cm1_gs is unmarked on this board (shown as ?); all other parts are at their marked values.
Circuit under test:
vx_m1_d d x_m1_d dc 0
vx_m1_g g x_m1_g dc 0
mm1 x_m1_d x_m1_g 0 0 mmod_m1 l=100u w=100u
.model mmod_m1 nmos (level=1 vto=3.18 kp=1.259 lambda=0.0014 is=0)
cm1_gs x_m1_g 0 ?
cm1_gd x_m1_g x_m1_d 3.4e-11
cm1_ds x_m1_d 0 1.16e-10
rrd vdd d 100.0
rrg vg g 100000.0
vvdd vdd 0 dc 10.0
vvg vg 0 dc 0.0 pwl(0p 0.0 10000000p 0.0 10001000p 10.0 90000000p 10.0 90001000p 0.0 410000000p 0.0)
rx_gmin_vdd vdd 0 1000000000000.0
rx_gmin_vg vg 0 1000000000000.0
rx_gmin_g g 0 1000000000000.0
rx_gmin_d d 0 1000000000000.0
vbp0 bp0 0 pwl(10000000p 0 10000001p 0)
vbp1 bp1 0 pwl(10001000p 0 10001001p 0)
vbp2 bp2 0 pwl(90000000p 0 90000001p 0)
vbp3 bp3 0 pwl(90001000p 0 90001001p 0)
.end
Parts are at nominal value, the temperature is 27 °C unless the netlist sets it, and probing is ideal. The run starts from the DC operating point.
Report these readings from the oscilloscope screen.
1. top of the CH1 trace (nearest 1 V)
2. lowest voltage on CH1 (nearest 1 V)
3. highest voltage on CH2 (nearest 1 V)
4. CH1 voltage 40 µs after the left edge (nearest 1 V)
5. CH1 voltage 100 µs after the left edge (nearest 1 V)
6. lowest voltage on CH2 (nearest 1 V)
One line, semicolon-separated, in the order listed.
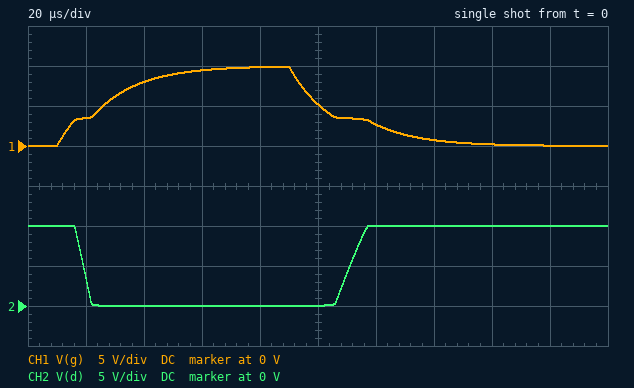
10 V; 0 V; 10 V; 8 V; 5 V; 0 V
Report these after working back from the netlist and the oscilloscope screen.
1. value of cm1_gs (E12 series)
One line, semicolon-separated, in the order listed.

120 pF
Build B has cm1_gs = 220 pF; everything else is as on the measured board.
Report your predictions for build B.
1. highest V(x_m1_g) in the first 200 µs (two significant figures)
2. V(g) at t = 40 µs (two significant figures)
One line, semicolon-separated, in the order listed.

9.5 V; 6.2 V
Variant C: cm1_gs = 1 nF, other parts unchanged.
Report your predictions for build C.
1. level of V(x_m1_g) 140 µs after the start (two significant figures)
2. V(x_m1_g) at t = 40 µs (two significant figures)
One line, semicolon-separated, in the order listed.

3.4 V; 2.5 V
